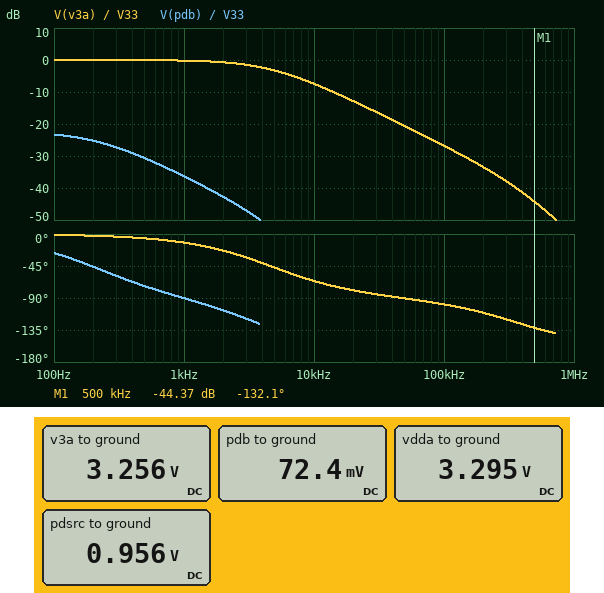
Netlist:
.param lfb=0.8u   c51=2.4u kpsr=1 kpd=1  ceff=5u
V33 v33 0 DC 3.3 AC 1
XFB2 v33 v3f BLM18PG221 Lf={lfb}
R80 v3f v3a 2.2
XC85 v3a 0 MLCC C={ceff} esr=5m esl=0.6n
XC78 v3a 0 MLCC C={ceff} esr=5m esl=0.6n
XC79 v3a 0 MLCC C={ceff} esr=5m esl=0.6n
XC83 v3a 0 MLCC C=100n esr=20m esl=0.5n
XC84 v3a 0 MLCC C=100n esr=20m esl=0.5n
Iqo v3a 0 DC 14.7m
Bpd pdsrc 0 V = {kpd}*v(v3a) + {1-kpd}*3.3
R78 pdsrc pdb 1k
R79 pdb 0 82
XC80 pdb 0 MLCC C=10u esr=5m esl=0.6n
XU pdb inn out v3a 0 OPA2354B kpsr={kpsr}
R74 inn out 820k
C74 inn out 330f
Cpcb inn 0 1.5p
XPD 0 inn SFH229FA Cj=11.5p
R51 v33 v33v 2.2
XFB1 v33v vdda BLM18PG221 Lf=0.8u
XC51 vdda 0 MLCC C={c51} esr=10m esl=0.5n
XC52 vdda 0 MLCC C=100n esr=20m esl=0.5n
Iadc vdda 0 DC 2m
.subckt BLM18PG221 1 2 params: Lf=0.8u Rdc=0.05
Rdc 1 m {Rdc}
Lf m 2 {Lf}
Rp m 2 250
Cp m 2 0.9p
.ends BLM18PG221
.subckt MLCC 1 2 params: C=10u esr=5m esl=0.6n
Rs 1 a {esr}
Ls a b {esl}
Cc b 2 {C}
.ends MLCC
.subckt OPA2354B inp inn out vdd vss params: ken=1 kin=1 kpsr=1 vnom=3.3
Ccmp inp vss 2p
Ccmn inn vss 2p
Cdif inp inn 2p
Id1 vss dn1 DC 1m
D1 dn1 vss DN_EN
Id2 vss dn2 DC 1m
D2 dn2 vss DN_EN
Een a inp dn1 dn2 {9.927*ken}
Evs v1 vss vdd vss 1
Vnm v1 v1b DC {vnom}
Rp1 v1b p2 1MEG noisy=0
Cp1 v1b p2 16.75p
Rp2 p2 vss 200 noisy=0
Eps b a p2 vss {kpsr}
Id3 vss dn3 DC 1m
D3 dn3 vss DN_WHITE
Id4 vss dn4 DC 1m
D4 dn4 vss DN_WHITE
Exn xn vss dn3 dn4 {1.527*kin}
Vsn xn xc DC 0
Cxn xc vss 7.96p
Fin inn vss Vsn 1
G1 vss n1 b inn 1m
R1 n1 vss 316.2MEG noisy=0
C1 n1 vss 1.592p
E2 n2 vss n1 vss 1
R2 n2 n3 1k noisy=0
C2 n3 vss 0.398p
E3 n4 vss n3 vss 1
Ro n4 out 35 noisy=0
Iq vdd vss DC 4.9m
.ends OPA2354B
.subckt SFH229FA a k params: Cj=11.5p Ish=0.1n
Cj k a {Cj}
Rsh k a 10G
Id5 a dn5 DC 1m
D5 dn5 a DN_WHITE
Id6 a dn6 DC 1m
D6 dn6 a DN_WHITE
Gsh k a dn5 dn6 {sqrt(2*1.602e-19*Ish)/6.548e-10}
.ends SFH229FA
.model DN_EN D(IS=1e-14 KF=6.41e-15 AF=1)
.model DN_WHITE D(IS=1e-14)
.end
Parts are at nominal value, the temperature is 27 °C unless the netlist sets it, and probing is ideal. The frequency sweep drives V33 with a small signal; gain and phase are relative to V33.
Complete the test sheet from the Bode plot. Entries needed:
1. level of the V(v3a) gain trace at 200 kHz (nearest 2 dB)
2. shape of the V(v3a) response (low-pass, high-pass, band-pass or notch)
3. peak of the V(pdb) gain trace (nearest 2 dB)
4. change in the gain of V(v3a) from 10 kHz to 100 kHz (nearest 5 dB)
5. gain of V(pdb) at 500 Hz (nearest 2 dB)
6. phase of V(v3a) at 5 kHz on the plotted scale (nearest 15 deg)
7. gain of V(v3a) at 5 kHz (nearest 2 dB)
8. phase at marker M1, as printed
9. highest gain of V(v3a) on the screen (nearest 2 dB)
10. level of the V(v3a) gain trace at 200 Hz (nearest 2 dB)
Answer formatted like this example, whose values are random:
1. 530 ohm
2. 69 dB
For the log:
1. -34 dB
2. low-pass
3. -24 dB
4. -20 dB
5. -30 dB
6. -45 deg
7. -4 dB
8. -132.1 deg
9. 0 dB
10. 0 dB
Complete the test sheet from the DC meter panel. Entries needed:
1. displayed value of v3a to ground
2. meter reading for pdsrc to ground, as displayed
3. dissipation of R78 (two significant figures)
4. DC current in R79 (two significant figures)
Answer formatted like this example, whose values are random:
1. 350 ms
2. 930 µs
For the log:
1. 3.256 V
2. 0.956 V
3. 780 µW
4. 880 µA
